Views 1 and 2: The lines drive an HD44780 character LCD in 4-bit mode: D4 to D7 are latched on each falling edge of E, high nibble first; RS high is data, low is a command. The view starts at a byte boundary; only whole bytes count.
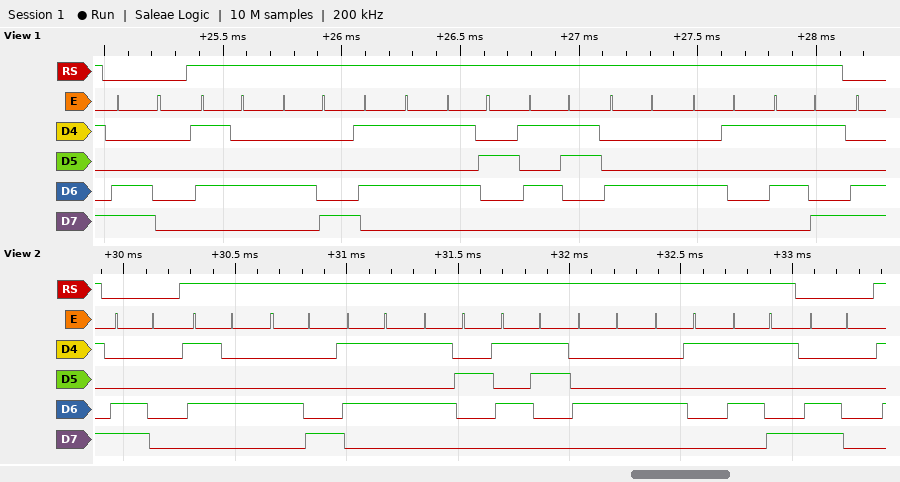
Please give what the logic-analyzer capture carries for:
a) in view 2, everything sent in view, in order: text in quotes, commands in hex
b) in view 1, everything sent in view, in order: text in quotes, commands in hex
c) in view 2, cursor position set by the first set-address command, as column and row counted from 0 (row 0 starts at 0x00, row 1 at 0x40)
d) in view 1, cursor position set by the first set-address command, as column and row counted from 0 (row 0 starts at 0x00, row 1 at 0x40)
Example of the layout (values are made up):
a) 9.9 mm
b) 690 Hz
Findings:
a) 0xC0 "THURSDAY" 0xC0
b) 0xC0 "THURSDAY"
c) column 0, row 1
d) column 0, row 1
